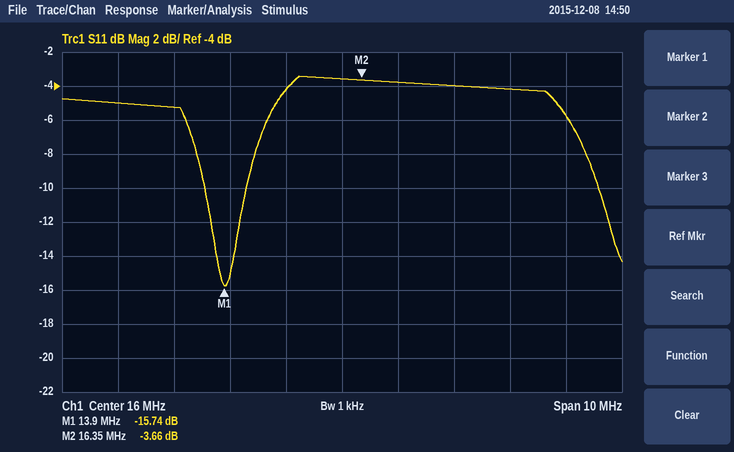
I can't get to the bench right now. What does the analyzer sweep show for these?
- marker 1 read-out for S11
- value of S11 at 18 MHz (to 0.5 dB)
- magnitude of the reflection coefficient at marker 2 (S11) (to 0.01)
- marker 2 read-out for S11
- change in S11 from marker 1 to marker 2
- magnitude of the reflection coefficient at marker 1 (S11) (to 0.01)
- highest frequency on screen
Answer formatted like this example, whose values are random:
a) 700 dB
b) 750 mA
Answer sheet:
a) -15.74 dB
b) -4.0 dB
c) 0.66
d) -3.66 dB
e) 12.08 dB
f) 0.16
g) 21 MHz
